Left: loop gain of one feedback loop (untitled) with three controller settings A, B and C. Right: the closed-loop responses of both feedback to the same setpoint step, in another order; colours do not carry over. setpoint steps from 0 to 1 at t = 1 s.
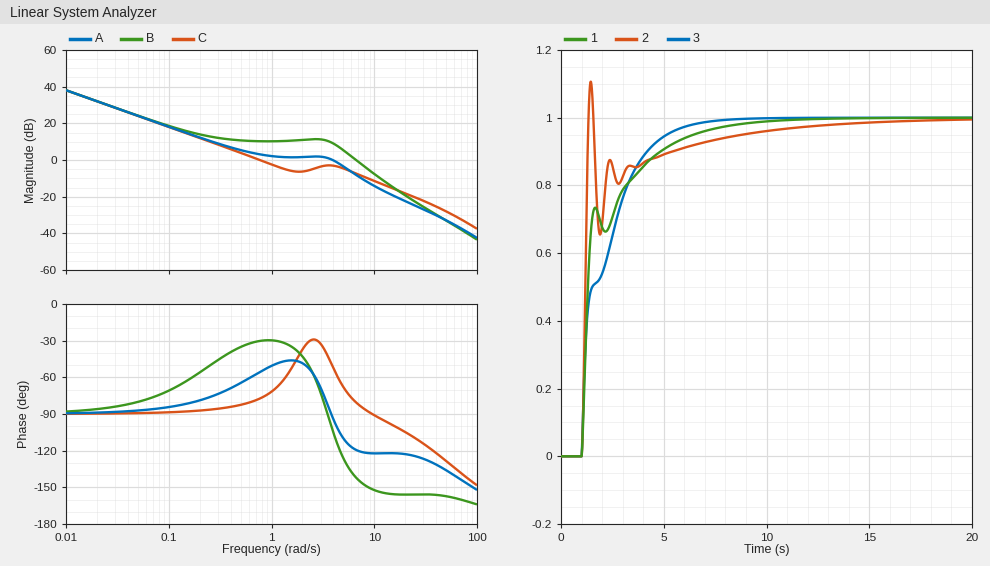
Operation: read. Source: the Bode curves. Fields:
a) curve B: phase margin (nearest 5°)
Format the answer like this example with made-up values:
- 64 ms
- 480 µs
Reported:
- 40°
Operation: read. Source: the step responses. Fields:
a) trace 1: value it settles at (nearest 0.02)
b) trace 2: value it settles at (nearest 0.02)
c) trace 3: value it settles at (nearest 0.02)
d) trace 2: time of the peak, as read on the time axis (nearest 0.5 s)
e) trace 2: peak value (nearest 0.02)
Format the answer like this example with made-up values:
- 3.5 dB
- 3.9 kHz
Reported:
- 1.00
- 1.00
- 1.00
- 1.5 s
- 1.10
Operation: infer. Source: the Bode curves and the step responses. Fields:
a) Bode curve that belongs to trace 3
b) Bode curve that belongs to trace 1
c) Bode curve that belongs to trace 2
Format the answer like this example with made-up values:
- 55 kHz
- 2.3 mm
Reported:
- C
- A
- B
